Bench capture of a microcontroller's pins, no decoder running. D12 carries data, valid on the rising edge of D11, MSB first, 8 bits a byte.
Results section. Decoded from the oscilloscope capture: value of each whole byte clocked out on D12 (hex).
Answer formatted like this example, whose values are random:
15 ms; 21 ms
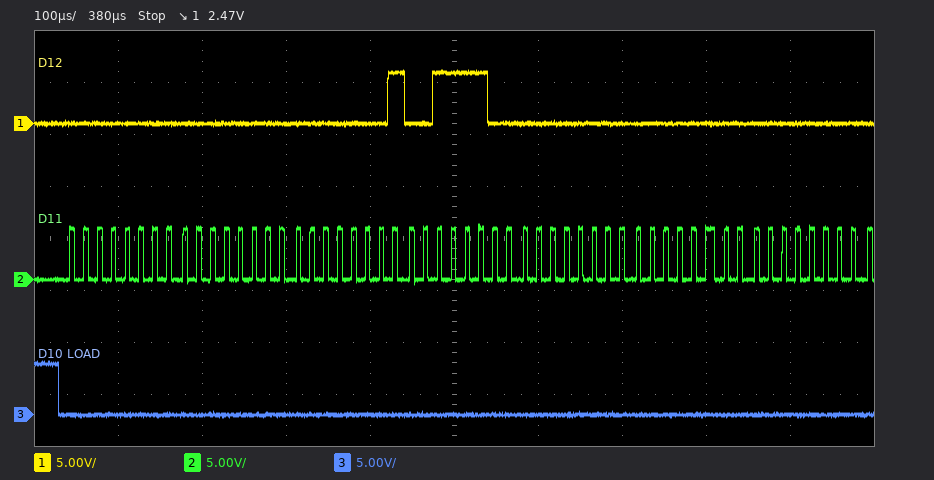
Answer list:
00 00 01 3C 00 00 00
